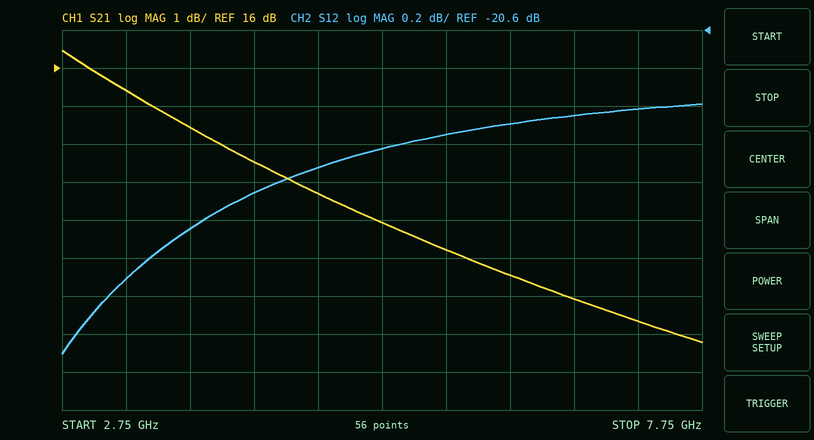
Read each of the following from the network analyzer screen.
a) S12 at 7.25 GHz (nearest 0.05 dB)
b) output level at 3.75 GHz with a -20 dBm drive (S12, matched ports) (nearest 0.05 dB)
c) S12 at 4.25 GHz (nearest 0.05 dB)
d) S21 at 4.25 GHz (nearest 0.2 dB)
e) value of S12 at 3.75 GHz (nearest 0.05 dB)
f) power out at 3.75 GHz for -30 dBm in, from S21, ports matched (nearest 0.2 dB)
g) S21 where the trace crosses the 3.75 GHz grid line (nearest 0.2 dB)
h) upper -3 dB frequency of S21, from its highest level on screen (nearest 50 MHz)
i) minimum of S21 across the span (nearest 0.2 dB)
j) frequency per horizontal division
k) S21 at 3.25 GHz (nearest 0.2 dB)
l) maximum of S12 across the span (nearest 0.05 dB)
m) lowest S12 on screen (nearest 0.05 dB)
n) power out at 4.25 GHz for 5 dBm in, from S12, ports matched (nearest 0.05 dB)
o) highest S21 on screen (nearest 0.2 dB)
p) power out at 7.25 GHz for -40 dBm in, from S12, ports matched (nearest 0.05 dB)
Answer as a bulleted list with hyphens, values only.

- -21.00 dB
- -41.65 dBm
- -21.45 dB
- 13.6 dB
- -21.65 dB
- -15.6 dBm
- 14.4 dB
- 4.30 GHz
- 8.8 dB
- 500 MHz
- 15.4 dB
- -21.00 dB
- -22.30 dB
- -16.45 dBm
- 16.4 dB
- -61.00 dBm
